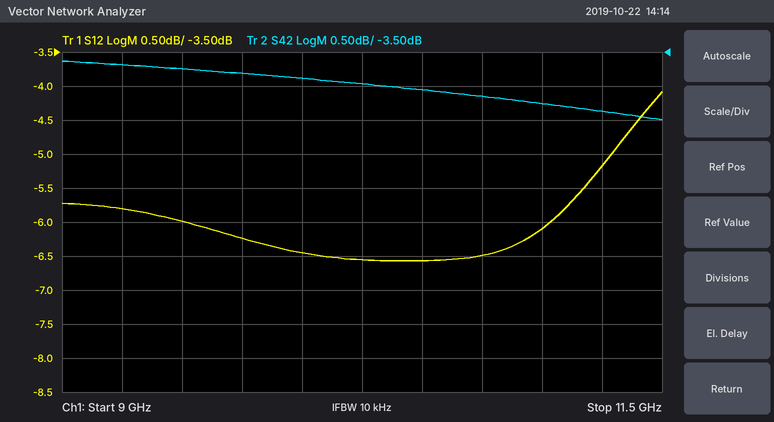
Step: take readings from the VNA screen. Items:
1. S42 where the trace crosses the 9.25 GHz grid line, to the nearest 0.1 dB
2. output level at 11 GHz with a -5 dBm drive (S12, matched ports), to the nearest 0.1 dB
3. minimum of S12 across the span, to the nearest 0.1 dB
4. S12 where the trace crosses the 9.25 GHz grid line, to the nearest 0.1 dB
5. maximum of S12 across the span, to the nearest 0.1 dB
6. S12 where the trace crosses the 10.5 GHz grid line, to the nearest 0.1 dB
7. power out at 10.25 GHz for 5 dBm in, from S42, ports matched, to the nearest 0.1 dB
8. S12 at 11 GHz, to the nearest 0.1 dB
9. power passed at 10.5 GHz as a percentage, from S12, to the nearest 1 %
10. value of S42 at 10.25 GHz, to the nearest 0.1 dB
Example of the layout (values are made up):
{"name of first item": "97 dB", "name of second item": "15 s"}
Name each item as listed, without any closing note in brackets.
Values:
{"S42 where the trace crosses the 9.25 GHz grid line, to the nearest 0.1 dB": "-3.7 dB", "output level at 11 GHz with a -5 dBm drive (S12, matched ports), to the nearest 0.1 dB": "-11.1 dBm", "minimum of S12 across the span, to the nearest 0.1 dB": "-6.6 dB", "S12 where the trace crosses the 9.25 GHz grid line, to the nearest 0.1 dB": "-5.8 dB", "maximum of S12 across the span, to the nearest 0.1 dB": "-4.1 dB", "S12 where the trace crosses the 10.5 GHz grid line, to the nearest 0.1 dB": "-6.6 dB", "power out at 10.25 GHz for 5 dBm in, from S42, ports matched, to the nearest 0.1 dB": "1.0 dBm", "S12 at 11 GHz, to the nearest 0.1 dB": "-6.1 dB", "power passed at 10.5 GHz as a percentage, from S12, to the nearest 1 %": "22 %", "value of S42 at 10.25 GHz, to the nearest 0.1 dB": "-4.0 dB"}
